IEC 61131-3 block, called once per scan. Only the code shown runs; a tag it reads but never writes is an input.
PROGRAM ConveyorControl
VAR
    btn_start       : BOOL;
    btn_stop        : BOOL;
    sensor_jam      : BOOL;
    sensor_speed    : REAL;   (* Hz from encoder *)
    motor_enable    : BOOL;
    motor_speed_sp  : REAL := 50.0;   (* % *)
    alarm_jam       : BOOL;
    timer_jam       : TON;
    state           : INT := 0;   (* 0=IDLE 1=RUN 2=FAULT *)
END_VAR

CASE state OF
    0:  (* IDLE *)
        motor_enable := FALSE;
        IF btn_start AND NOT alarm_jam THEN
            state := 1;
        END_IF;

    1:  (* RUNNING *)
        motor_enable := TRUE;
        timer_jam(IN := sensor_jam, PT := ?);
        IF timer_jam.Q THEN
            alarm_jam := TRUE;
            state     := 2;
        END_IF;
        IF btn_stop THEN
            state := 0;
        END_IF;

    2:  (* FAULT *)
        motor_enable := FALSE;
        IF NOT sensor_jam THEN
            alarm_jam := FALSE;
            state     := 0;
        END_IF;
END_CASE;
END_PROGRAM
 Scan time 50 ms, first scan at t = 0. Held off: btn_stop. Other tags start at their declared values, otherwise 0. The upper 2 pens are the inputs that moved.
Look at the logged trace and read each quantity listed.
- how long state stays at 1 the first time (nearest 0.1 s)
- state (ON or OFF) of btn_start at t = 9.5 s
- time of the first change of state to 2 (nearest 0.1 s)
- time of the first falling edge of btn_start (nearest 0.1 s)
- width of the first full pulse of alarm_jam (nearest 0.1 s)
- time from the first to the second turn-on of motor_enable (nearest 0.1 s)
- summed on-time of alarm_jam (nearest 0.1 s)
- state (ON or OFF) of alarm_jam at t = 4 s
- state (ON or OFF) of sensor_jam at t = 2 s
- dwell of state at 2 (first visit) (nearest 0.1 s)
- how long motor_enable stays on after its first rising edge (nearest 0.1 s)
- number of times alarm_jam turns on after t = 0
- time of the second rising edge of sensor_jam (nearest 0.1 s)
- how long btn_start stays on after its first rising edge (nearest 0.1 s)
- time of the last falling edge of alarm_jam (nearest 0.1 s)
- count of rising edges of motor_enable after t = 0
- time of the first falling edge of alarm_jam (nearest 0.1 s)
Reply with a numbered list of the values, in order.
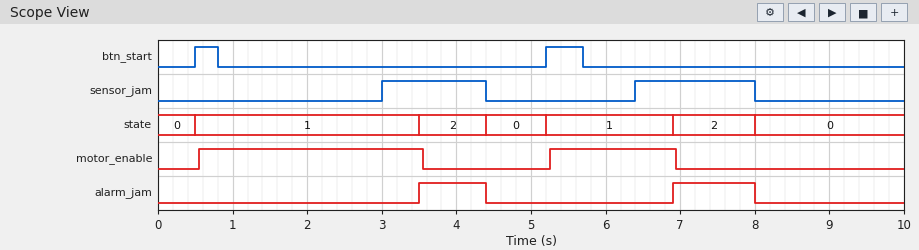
1. 3.0 s
2. OFF
3. 3.5 s
4. 0.8 s
5. 0.9 s
6. 4.7 s
7. 2.0 s
8. ON
9. OFF
10. 0.9 s
11. 3.0 s
12. 2
13. 6.4 s
14. 0.3 s
15. 8.0 s
16. 2
17. 4.4 s
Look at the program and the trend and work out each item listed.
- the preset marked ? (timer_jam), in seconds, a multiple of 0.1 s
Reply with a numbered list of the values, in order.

1. 0.5 s
